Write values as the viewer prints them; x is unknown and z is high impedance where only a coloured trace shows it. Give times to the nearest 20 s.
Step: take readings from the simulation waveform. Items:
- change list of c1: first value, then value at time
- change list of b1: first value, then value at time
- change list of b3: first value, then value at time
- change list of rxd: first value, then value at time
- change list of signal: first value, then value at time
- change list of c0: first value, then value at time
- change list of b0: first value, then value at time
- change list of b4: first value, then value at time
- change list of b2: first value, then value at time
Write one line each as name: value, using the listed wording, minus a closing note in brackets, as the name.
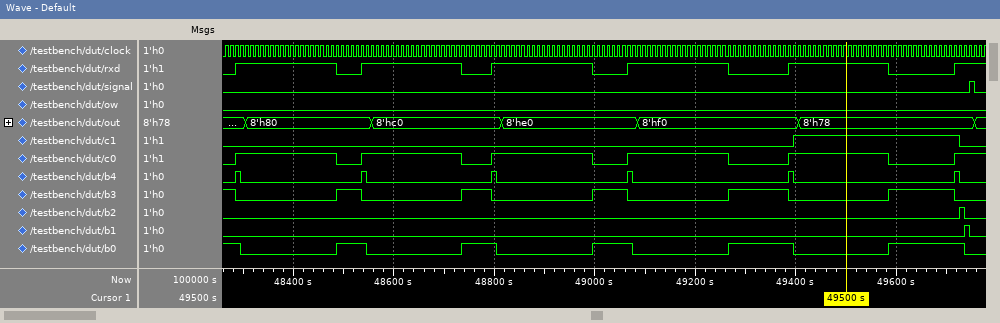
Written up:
change list of c1: first value, then value at time: 0, 1 at 49400 s, 0 at 49720 s
change list of b1: first value, then value at time: 0, 1 at 49740 s, 0 at 49740 s
change list of b3: first value, then value at time: 1, 0 at 48280 s, 1 at 48480 s, 0 at 48540 s, 1 at 48740 s, 0 at 48800 s, 1 at 49000 s, 0 at 49060 s, 1 at 49260 s, 0 at 49380 s, 1 at 49580 s, 0 at 49720 s
change list of rxd: first value, then value at time: 0, 1 at 48280 s, 0 at 48480 s, 1 at 48540 s, 0 at 48740 s, 1 at 48800 s, 0 at 49000 s, 1 at 49060 s, 0 at 49260 s, 1 at 49380 s, 0 at 49580 s, 1 at 49720 s
change list of signal: first value, then value at time: 0, 1 at 49740 s, 0 at 49760 s
change list of c0: first value, then value at time: 0, 1 at 48280 s, 0 at 48480 s, 1 at 48540 s, 0 at 48740 s, 1 at 48800 s, 0 at 49000 s, 1 at 49060 s, 0 at 49260 s, 1 at 49380 s, 0 at 49580 s, 1 at 49720 s
change list of b0: first value, then value at time: 1, 0 at 48300 s, 1 at 48480 s, 0 at 48540 s, 1 at 48740 s, 0 at 48800 s, 1 at 49000 s, 0 at 49080 s, 1 at 49260 s, 0 at 49400 s, 1 at 49580 s, 0 at 49740 s
change list of b4: first value, then value at time: 0, 1 at 48280 s, 0 at 48300 s, 1 at 48540 s, 0 at 48540 s, 1 at 48800 s, 0 at 48800 s, 1 at 49060 s, 0 at 49080 s, 1 at 49380 s, 0 at 49400 s, 1 at 49720 s, 0 at 49720 s
change list of b2: first value, then value at time: 0, 1 at 49720 s, 0 at 49740 s
